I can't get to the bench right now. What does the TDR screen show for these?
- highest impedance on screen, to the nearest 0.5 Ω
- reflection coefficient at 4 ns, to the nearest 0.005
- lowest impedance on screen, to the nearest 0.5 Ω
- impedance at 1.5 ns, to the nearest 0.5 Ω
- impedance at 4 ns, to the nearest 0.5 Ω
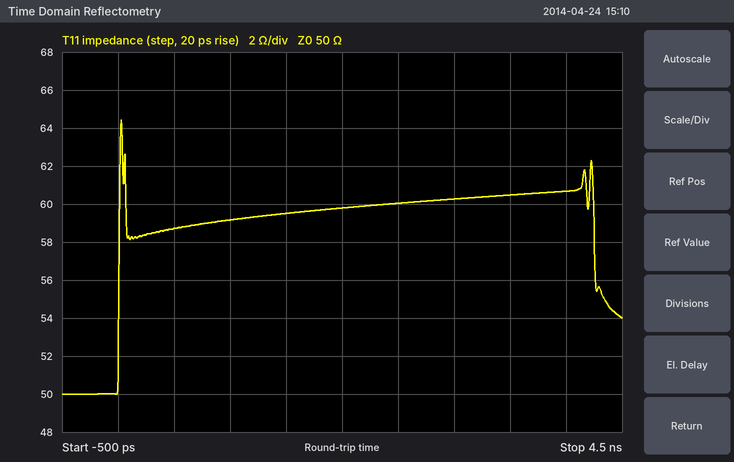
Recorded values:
64.5 Ω
+0.095
50.0 Ω
59.5 Ω
60.5 Ω
